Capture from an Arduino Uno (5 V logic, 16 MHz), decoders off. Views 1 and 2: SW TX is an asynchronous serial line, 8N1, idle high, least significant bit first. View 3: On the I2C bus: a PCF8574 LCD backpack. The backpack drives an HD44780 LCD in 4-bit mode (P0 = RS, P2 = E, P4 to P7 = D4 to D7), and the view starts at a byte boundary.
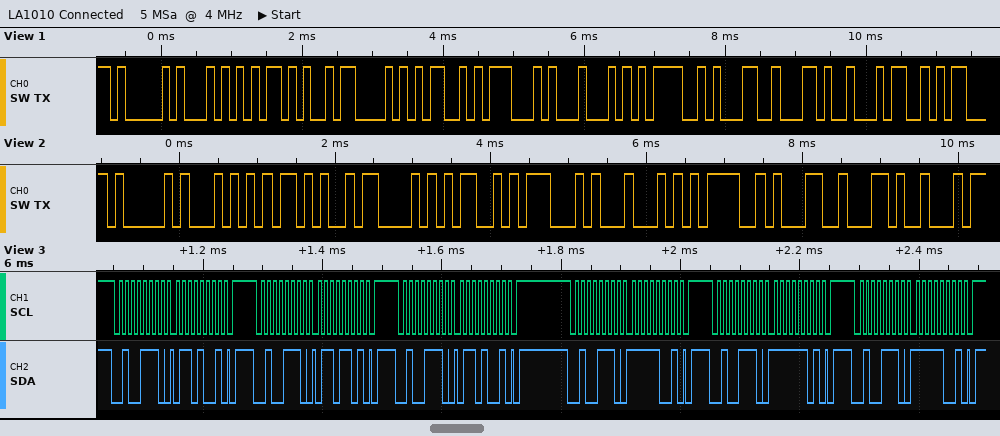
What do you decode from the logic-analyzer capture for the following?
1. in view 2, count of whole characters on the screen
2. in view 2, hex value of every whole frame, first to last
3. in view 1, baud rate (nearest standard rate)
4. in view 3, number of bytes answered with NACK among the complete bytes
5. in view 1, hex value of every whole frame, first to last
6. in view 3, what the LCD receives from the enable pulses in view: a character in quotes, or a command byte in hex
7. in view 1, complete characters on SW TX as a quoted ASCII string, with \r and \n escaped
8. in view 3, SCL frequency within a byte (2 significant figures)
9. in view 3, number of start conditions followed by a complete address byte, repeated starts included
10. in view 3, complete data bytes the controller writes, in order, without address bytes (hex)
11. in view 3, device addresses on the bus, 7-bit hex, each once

10
41 54 2B 43 4D 47 44 3D 31 2C
9600 baud
0
0x41 0x54 0x2B 0x43 0x4D 0x47 0x44 0x3D 0x31 0x2C 0x34
'o'
"AT+CMGD=1,4"
100 kHz
6
69 6D 69 F9 FD F9
0x27
